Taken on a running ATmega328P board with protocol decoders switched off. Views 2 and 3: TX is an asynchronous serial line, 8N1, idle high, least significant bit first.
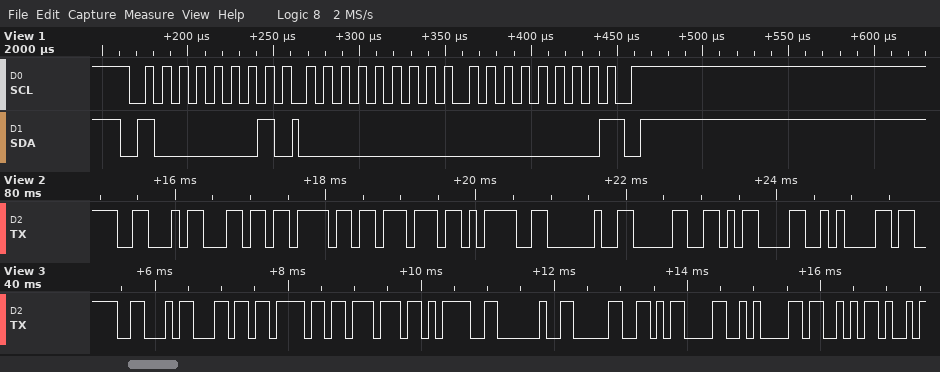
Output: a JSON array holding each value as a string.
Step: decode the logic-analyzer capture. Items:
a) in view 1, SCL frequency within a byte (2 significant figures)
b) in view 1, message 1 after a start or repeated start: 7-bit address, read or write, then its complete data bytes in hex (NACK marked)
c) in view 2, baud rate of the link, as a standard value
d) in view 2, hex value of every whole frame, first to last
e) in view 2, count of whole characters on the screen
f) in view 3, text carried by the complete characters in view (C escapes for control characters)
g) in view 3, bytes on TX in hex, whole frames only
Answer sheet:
["100 kHz", "0x40 read: 00 00 NACK", "9600 baud", "46 6C 6F 77 3D 20 30 0D 0A", "9", "\"Flow= 0\\r\\nS\"", "46 6C 6F 77 3D 20 30 0D 0A 53"]
